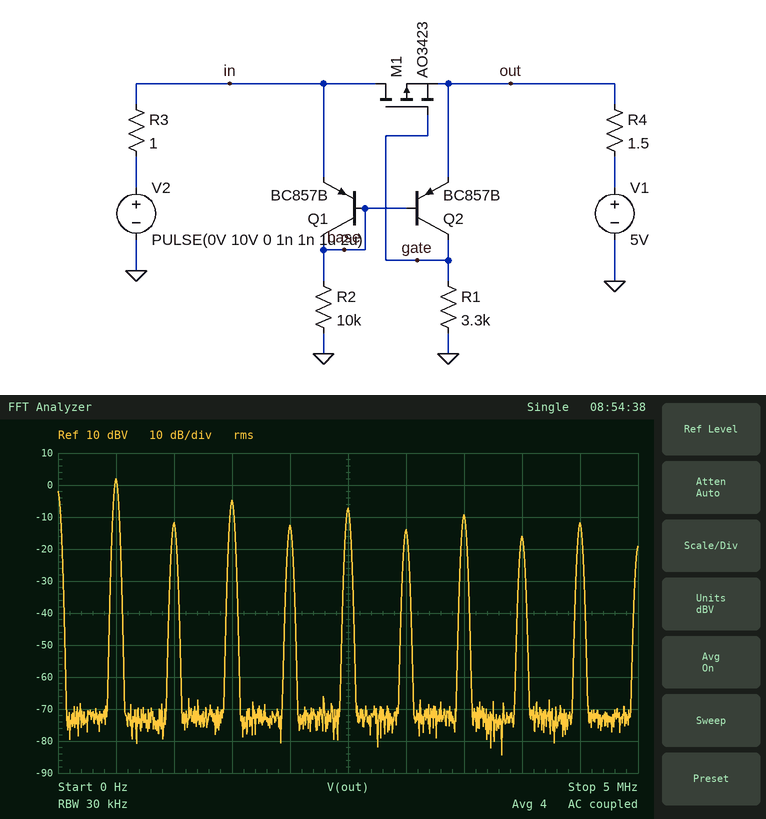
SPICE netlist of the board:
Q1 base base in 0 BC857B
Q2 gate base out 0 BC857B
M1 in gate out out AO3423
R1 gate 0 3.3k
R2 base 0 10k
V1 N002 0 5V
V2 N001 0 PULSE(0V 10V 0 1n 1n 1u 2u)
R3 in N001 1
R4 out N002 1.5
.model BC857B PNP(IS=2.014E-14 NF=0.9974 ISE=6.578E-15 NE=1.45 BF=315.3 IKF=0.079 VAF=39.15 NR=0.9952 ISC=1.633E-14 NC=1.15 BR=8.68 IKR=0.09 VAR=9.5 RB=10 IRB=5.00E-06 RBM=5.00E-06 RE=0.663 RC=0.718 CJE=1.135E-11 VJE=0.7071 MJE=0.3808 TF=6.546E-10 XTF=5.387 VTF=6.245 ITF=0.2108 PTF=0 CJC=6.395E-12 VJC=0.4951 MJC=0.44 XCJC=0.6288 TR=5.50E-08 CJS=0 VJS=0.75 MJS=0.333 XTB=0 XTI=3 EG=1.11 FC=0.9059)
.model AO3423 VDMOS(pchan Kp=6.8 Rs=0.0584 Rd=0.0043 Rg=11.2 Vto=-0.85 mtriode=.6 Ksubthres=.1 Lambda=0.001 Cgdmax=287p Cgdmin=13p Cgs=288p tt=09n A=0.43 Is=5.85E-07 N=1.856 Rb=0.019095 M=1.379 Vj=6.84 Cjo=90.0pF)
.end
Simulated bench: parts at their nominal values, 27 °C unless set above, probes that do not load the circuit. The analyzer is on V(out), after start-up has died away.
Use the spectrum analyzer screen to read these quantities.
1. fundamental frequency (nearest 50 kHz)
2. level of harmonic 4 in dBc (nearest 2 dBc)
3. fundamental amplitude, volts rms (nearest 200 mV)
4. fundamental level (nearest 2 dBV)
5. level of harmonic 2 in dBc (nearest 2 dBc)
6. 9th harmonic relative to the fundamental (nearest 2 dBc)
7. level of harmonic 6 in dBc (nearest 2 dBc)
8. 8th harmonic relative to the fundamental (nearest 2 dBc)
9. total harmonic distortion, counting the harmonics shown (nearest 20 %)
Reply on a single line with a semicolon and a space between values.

500 kHz; -14 dBc; 1.2 V; 2 dBV; -14 dBc; -14 dBc; -16 dBc; -18 dBc; 80 %
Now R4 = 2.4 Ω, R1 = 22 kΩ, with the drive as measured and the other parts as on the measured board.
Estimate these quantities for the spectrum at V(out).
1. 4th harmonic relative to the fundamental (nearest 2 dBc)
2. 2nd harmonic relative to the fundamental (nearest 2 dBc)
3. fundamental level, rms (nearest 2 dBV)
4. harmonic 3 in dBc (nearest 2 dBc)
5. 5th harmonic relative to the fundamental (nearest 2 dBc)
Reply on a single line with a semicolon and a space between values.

-38 dBc; -38 dBc; 2 dBV; -10 dBc; -14 dBc
